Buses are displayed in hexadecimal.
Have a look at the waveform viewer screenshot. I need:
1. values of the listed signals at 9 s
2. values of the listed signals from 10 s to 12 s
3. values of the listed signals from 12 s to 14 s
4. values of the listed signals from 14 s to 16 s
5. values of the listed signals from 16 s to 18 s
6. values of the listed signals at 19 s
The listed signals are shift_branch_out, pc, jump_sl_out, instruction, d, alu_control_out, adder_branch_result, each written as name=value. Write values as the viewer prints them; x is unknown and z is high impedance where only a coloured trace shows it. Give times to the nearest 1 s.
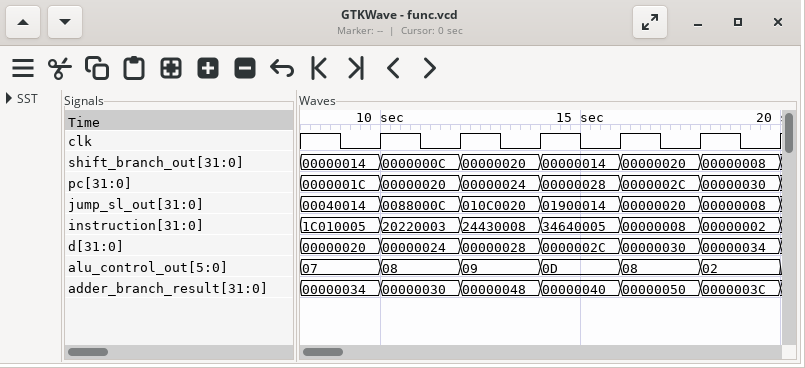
shift_branch_out=00000014, pc=0000001C, jump_sl_out=00040014, instruction=1C010005, d=00000020, alu_control_out=07, adder_branch_result=00000034
shift_branch_out=0000000C, pc=00000020, jump_sl_out=0088000C, instruction=20220003, d=00000024, alu_control_out=08, adder_branch_result=00000030
shift_branch_out=00000020, pc=00000024, jump_sl_out=010C0020, instruction=24430008, d=00000028, alu_control_out=09, adder_branch_result=00000048
shift_branch_out=00000014, pc=00000028, jump_sl_out=01900014, instruction=34640005, d=0000002C, alu_control_out=0D, adder_branch_result=00000040
shift_branch_out=00000020, pc=0000002C, jump_sl_out=00000020, instruction=00000008, d=00000030, alu_control_out=08, adder_branch_result=00000050
shift_branch_out=00000008, pc=00000030, jump_sl_out=00000008, instruction=00000002, d=00000034, alu_control_out=02, adder_branch_result=0000003C
